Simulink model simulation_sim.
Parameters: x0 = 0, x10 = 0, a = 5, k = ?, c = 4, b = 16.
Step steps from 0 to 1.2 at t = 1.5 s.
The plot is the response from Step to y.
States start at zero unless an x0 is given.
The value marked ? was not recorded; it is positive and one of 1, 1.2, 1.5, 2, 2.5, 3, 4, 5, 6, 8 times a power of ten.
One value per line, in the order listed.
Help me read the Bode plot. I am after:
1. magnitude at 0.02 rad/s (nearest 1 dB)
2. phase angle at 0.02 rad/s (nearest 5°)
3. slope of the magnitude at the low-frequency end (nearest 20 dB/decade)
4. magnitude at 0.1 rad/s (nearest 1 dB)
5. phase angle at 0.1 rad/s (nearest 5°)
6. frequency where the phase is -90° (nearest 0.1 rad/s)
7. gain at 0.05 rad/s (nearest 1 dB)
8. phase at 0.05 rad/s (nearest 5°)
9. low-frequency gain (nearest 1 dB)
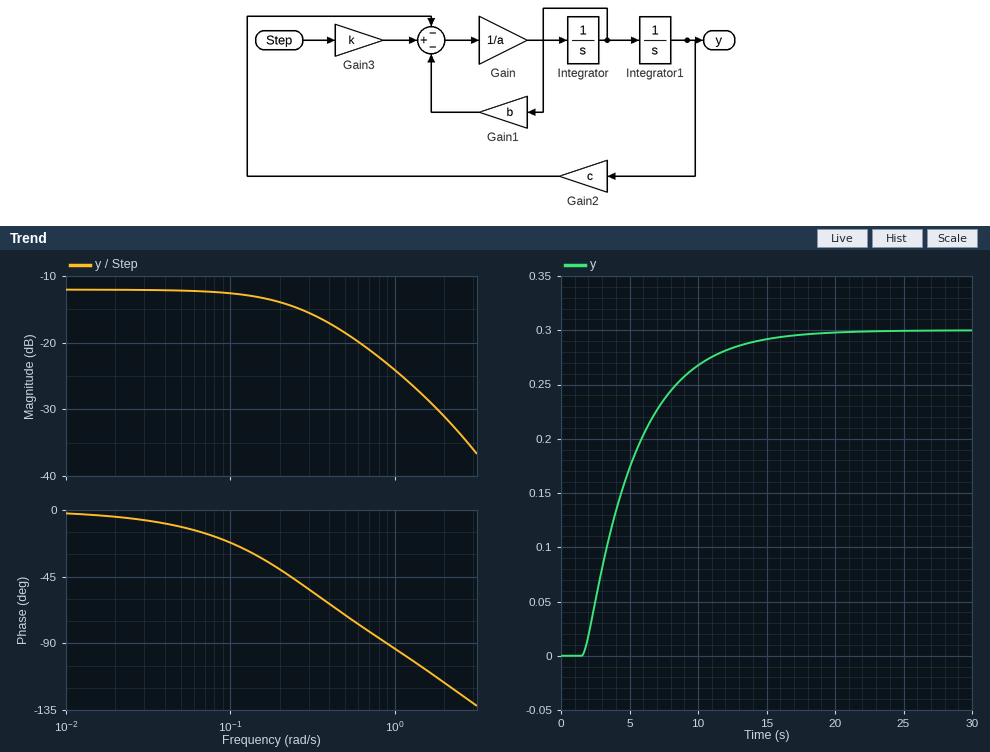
-12 dB
-5°
0 dB/decade
-13 dB
-20°
0.9 rad/s
-12 dB
-10°
-12 dB
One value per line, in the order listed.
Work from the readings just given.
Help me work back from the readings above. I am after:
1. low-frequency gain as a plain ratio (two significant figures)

0.25
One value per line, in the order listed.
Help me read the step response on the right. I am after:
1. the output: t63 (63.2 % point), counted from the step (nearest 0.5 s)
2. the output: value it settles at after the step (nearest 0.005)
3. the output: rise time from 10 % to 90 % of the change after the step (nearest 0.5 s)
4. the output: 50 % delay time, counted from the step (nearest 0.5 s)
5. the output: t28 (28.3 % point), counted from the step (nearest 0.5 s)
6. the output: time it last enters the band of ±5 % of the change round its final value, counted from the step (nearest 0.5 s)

4.0 s
0.300
8.0 s
3.0 s
1.5 s
11.5 s
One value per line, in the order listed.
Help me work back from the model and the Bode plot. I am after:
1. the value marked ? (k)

1
